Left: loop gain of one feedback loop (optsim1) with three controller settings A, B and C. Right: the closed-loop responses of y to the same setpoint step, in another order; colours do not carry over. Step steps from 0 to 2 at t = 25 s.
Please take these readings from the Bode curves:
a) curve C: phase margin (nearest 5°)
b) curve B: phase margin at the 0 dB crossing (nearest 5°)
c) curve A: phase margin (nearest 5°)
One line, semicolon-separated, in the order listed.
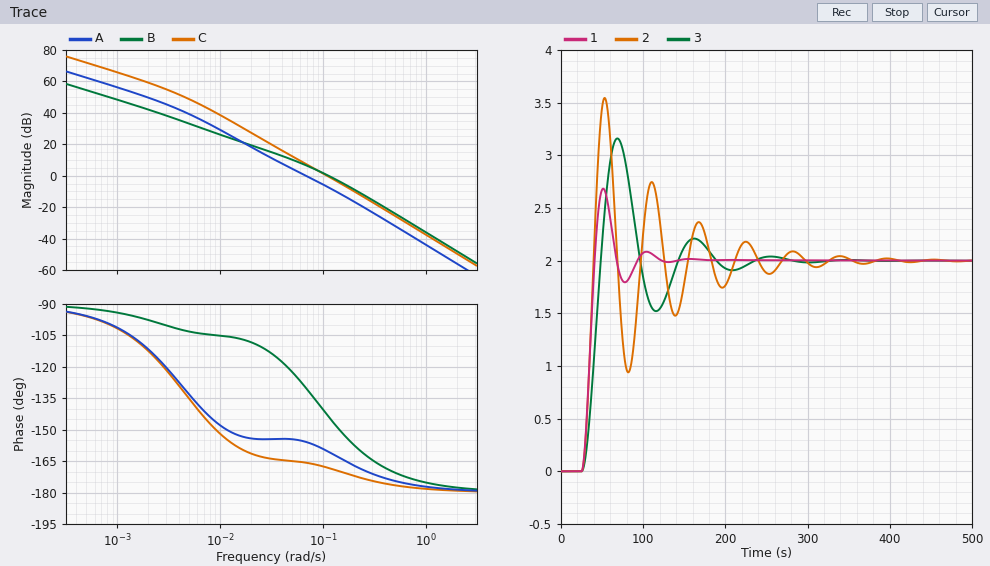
10°; 35°; 25°
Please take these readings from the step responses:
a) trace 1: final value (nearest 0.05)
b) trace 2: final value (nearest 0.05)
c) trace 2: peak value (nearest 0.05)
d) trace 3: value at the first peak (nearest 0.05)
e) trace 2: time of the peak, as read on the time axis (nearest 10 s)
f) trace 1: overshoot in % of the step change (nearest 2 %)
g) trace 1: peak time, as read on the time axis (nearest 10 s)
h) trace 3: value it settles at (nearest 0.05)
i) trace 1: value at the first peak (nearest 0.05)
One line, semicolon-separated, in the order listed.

2.00; 2.00; 3.55; 3.15; 50 s; 34 %; 50 s; 2.00; 2.70
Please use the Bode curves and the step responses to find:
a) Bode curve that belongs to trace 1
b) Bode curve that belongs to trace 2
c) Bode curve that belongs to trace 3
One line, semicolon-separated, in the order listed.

B; C; A
